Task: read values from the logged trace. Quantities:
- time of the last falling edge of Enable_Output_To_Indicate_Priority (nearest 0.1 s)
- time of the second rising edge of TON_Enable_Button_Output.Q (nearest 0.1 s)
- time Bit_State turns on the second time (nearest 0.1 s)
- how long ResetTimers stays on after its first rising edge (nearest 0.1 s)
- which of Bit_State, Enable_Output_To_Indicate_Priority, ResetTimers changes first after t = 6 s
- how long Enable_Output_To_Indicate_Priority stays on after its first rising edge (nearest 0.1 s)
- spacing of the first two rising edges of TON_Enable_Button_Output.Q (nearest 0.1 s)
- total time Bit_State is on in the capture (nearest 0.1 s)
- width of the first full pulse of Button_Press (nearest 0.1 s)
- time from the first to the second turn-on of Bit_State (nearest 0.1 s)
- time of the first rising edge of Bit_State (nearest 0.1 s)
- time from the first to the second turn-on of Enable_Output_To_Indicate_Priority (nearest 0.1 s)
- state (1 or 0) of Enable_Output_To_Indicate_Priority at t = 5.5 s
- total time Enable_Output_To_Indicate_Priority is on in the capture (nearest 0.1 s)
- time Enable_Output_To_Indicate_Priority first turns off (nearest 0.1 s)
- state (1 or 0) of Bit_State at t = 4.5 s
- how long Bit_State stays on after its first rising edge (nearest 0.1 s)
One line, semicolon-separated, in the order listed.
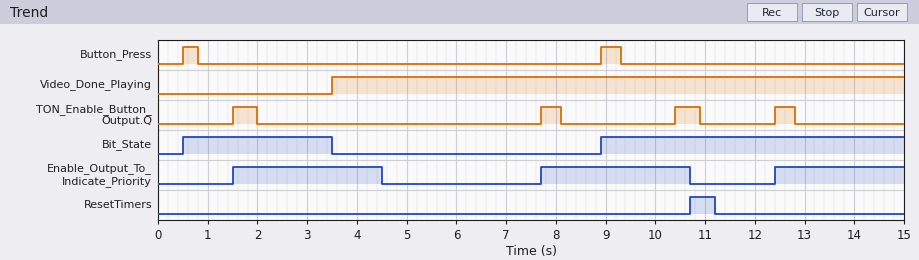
10.7 s; 7.7 s; 8.9 s; 0.5 s; Enable_Output_To_Indicate_Priority; 3.0 s; 6.2 s; 9.1 s; 0.3 s; 8.4 s; 0.5 s; 6.2 s; 0; 8.6 s; 4.5 s; 0; 3.0 s
